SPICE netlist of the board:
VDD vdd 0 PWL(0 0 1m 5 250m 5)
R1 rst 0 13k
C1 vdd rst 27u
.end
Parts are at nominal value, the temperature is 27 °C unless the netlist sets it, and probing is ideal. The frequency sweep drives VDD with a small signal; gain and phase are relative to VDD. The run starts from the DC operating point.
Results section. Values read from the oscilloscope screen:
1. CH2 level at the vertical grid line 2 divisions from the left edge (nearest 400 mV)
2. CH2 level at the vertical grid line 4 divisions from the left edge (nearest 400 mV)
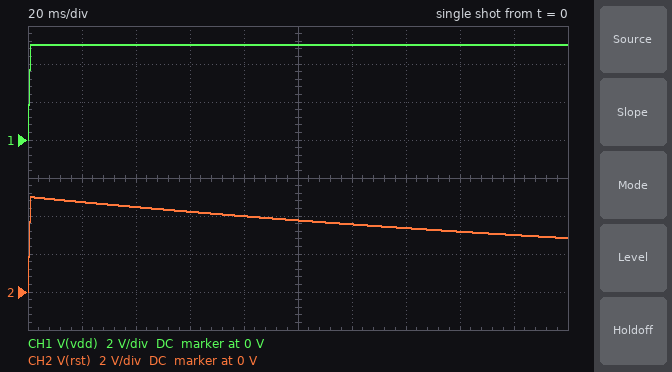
4.4 V
4.0 V
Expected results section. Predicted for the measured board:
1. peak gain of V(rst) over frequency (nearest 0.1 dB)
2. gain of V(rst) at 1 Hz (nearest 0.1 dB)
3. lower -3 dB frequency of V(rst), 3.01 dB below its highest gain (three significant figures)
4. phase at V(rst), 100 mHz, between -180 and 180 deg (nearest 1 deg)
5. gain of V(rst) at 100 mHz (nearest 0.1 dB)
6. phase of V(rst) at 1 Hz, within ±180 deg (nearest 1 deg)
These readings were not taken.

0 dB
-0.8 dB
453 mHz
78 deg
-13.3 dB
24 deg
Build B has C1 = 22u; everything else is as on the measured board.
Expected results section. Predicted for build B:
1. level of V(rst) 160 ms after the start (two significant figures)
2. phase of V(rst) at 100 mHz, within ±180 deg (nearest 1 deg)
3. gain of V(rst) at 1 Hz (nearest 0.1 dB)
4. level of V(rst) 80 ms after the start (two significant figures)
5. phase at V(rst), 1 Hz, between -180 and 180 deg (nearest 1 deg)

2.9 V
80 deg
-1.2 dB
3.8 V
29 deg
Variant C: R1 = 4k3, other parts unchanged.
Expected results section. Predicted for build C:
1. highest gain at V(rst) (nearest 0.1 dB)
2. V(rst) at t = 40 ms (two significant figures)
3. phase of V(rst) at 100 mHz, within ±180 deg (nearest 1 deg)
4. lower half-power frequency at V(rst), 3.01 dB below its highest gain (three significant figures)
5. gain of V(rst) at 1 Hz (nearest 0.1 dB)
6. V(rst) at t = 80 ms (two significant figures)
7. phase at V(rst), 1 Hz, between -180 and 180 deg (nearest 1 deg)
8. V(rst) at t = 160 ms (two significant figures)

0 dB
3.6 V
86 deg
1.37 Hz
-4.6 dB
2.5 V
54 deg
1.3 V
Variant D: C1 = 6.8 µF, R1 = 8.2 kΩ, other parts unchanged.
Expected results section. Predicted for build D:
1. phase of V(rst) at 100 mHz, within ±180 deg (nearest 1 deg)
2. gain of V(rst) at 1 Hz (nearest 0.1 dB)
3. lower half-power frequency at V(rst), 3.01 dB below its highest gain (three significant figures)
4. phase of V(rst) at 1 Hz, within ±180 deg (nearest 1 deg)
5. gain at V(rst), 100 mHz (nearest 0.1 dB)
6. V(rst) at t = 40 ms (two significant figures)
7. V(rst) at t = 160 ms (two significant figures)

88 deg
-9.6 dB
2.85 Hz
71 deg
-29.1 dB
2.5 V
290 mV
